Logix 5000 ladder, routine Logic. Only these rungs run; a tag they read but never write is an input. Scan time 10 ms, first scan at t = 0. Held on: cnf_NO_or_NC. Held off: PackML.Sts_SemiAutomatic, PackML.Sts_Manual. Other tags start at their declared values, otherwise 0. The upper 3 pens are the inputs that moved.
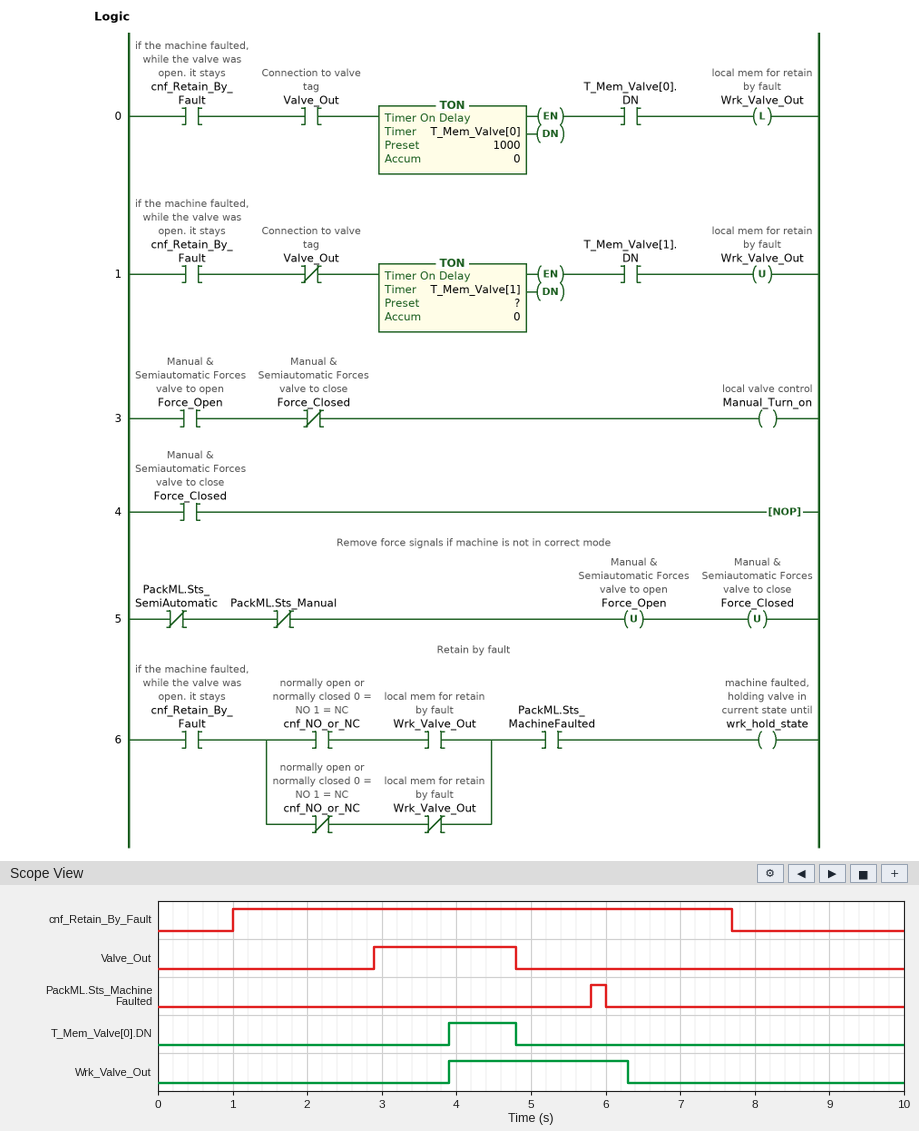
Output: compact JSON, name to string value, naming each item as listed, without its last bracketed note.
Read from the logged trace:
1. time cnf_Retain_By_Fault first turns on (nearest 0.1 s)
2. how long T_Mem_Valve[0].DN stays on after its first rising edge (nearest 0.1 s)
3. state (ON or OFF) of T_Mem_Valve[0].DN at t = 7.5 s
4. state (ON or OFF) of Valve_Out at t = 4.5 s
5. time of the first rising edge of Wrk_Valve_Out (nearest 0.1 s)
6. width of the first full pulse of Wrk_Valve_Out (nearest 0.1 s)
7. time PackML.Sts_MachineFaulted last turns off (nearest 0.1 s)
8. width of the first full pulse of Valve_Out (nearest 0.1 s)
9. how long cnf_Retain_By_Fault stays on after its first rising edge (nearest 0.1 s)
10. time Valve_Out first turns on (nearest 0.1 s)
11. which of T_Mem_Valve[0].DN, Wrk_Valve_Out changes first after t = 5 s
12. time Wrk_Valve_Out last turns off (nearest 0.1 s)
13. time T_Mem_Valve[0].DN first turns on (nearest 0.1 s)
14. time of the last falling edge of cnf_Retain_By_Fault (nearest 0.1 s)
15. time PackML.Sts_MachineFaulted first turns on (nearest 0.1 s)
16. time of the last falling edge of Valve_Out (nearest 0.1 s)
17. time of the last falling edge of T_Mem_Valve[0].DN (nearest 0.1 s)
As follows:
{"time cnf_Retain_By_Fault first turns on": "1.0 s", "how long T_Mem_Valve[0].DN stays on after its first rising edge": "0.9 s", "state (ON or OFF) of T_Mem_Valve[0].DN at t = 7.5 s": "OFF", "state (ON or OFF) of Valve_Out at t = 4.5 s": "ON", "time of the first rising edge of Wrk_Valve_Out": "3.9 s", "width of the first full pulse of Wrk_Valve_Out": "2.4 s", "time PackML.Sts_MachineFaulted last turns off": "6.0 s", "width of the first full pulse of Valve_Out": "1.9 s", "how long cnf_Retain_By_Fault stays on after its first rising edge": "6.7 s", "time Valve_Out first turns on": "2.9 s", "which of T_Mem_Valve[0].DN, Wrk_Valve_Out changes first after t = 5 s": "Wrk_Valve_Out", "time Wrk_Valve_Out last turns off": "6.3 s", "time T_Mem_Valve[0].DN first turns on": "3.9 s", "time of the last falling edge of cnf_Retain_By_Fault": "7.7 s", "time PackML.Sts_MachineFaulted first turns on": "5.8 s", "time of the last falling edge of Valve_Out": "4.8 s", "time of the last falling edge of T_Mem_Valve[0].DN": "4.8 s"}
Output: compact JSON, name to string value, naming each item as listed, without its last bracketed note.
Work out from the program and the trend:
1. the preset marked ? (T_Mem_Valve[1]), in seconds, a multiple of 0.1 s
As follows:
{"the preset marked ? (T_Mem_Valve[1]), in seconds, a multiple of 0.1 s": "1.5 s"}
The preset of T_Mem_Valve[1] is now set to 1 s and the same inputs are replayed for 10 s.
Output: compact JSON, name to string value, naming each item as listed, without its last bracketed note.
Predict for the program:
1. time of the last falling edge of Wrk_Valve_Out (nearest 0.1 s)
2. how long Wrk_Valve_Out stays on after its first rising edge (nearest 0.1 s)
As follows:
{"time of the last falling edge of Wrk_Valve_Out": "5.8 s", "how long Wrk_Valve_Out stays on after its first rising edge": "1.9 s"}
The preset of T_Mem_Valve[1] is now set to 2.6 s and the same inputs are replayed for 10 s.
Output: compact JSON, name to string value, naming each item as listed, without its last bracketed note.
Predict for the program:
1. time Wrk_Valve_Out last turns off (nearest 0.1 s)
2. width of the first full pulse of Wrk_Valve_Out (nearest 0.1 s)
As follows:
{"time Wrk_Valve_Out last turns off": "7.4 s", "width of the first full pulse of Wrk_Valve_Out": "3.5 s"}
